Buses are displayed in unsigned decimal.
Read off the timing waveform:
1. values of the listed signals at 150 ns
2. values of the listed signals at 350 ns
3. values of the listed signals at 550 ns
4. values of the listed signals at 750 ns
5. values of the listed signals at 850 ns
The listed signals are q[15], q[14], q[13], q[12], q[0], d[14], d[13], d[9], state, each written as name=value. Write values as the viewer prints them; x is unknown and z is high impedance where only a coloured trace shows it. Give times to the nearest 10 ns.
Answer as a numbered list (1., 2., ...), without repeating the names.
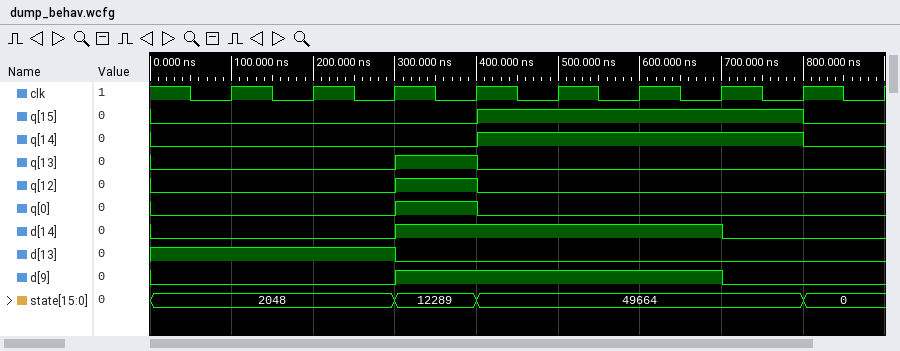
1. q[15]=0, q[14]=0, q[13]=0, q[12]=0, q[0]=0, d[14]=0, d[13]=1, d[9]=0, state=2048
2. q[15]=0, q[14]=0, q[13]=1, q[12]=1, q[0]=1, d[14]=1, d[13]=0, d[9]=1, state=12289
3. q[15]=1, q[14]=1, q[13]=0, q[12]=0, q[0]=0, d[14]=1, d[13]=0, d[9]=1, state=49664
4. q[15]=1, q[14]=1, q[13]=0, q[12]=0, q[0]=0, d[14]=0, d[13]=0, d[9]=0, state=49664
5. q[15]=0, q[14]=0, q[13]=0, q[12]=0, q[0]=0, d[14]=0, d[13]=0, d[9]=0, state=0
